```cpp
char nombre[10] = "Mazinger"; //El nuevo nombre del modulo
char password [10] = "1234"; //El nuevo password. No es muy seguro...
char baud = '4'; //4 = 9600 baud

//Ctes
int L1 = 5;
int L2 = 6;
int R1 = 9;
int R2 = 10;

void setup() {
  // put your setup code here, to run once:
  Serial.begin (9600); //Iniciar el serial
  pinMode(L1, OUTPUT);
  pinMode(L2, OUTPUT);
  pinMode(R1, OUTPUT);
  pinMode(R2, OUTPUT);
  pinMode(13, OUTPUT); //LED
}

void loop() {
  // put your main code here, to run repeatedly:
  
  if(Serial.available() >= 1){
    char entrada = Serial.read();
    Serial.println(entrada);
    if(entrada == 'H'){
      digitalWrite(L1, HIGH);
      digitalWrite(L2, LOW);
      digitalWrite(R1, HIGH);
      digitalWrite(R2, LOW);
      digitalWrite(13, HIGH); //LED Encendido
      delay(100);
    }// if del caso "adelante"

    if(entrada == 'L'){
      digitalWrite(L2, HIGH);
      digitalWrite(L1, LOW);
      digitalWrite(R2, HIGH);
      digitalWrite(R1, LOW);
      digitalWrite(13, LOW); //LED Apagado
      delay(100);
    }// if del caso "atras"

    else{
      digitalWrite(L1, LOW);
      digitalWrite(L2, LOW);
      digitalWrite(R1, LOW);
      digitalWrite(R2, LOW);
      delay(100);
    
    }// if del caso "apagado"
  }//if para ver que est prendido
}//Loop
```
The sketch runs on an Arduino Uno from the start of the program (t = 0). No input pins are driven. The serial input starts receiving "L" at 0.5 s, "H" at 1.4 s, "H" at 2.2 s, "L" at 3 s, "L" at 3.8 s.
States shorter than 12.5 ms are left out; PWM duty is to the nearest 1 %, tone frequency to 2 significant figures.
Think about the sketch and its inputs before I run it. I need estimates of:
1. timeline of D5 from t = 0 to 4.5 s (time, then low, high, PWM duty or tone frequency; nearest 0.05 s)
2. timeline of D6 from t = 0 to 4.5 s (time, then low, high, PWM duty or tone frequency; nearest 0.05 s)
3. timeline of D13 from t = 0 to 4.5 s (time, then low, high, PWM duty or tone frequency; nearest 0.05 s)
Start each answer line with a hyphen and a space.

- 0 s low; 1.4 s high; 1.5 s low; 2.2 s high; 2.3 s low
- 0 s low; 0.5 s high; 1.4 s low; 3 s high
- 0 s low; 1.4 s high; 3 s low
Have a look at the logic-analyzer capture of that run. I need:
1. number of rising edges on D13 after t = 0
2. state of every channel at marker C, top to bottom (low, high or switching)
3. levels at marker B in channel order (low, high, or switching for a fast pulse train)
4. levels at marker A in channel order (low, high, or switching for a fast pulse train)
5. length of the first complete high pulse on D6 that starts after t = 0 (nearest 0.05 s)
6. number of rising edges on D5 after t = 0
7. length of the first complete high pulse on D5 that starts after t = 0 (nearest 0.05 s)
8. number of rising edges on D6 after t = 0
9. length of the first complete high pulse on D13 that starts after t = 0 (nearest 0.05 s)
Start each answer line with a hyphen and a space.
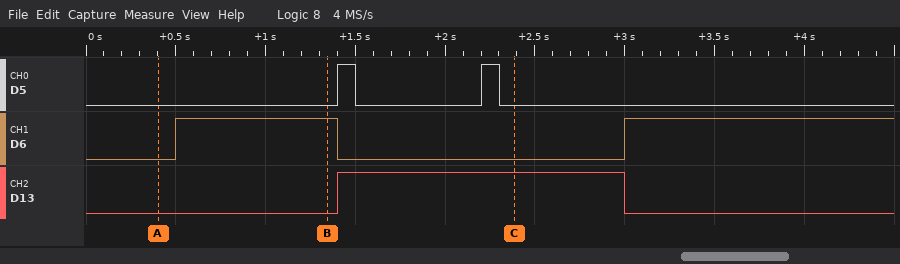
- 1
- D5 low, D6 low, D13 high
- D5 low, D6 high, D13 low
- D5 low, D6 low, D13 low
- 0.90 s
- 2
- 0.10 s
- 2
- 1.60 s
